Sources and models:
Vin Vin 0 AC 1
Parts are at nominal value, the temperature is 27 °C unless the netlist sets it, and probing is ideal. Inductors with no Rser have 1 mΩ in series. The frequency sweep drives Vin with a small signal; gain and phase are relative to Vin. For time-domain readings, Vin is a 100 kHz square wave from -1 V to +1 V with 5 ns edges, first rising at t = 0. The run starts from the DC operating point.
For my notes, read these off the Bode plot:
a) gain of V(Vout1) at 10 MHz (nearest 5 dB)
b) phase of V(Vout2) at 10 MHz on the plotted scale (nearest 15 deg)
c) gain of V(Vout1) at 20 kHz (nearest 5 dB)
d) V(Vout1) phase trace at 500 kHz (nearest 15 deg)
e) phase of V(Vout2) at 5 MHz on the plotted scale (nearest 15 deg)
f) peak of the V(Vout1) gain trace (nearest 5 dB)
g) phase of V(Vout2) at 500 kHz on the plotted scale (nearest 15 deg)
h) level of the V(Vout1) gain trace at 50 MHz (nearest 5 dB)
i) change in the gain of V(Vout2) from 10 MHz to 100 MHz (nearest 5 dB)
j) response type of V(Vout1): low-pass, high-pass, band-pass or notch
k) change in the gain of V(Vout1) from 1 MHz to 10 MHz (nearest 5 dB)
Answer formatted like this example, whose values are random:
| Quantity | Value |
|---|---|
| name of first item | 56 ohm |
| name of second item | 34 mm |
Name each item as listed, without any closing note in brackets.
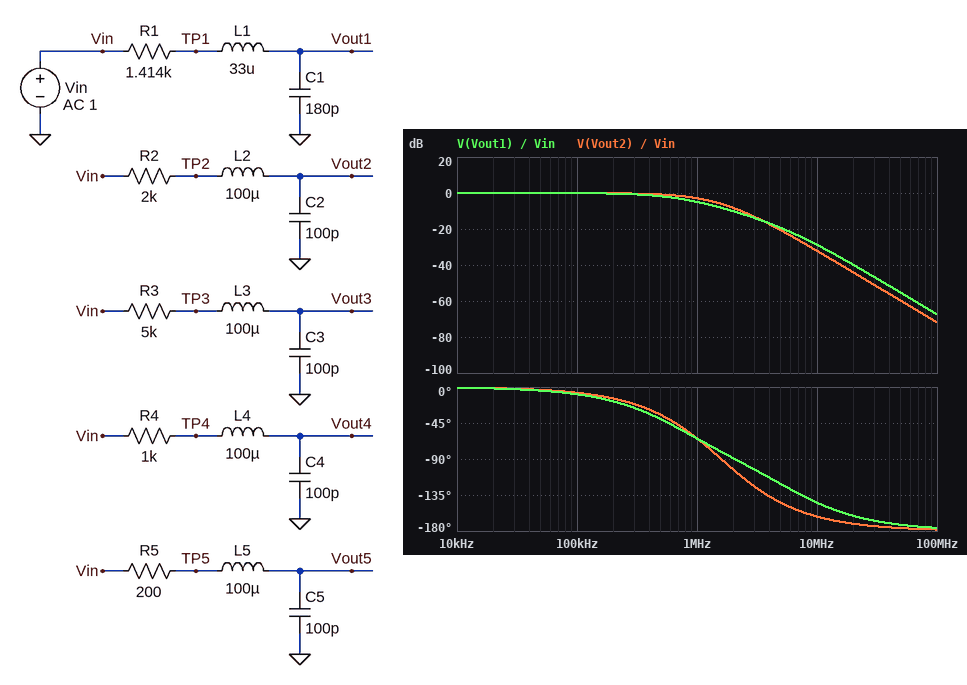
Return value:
| Quantity | Value |
|---|---|
| gain of V(Vout1) at 10 MHz | -30 dB |
| phase of V(Vout2) at 10 MHz on the plotted scale | -165 deg |
| gain of V(Vout1) at 20 kHz | 0 dB |
| V(Vout1) phase trace at 500 kHz | -45 deg |
| phase of V(Vout2) at 5 MHz on the plotted scale | -150 deg |
| peak of the V(Vout1) gain trace | 0 dB |
| phase of V(Vout2) at 500 kHz on the plotted scale | -30 deg |
| level of the V(Vout1) gain trace at 50 MHz | -55 dB |
| change in the gain of V(Vout2) from 10 MHz to 100 MHz | -40 dB |
| response type of V(Vout1): low-pass, high-pass, band-pass or notch | low-pass |
| change in the gain of V(Vout1) from 1 MHz to 10 MHz | -25 dB |
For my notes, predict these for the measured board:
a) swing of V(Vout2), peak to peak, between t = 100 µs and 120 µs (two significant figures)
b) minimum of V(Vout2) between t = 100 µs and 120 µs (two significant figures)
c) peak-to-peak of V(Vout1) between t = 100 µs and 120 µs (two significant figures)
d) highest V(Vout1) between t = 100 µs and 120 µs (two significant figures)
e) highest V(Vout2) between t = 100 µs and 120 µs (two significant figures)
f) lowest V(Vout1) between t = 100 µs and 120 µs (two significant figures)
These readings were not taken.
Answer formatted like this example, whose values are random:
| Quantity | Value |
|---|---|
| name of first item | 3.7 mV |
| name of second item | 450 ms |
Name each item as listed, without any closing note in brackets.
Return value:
| Quantity | Value |
|---|---|
| swing of V(Vout2), peak to peak, between t = 100 µs and 120 µs | 2.0 V |
| minimum of V(Vout2) between t = 100 µs and 120 µs | -1.0 V |
| peak-to-peak of V(Vout1) between t = 100 µs and 120 µs | 2.0 V |
| highest V(Vout1) between t = 100 µs and 120 µs | 1.0 V |
| highest V(Vout2) between t = 100 µs and 120 µs | 1.0 V |
| lowest V(Vout1) between t = 100 µs and 120 µs | -1.0 V |
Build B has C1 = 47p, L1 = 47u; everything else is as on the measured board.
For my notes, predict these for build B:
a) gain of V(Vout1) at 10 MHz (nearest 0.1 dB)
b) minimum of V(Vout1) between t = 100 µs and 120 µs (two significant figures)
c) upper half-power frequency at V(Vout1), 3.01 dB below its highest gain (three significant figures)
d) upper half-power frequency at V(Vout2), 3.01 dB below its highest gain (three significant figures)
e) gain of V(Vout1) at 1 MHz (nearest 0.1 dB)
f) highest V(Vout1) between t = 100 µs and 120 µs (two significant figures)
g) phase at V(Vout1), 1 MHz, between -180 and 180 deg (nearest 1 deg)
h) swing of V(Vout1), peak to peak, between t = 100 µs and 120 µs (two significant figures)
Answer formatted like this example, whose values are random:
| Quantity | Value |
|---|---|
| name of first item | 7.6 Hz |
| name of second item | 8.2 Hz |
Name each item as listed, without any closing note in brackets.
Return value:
| Quantity | Value |
|---|---|
| gain of V(Vout1) at 10 MHz | -18.9 dB |
| minimum of V(Vout1) between t = 100 µs and 120 µs | -1.1 V |
| upper half-power frequency at V(Vout1), 3.01 dB below its highest gain | 3.39 MHz |
| upper half-power frequency at V(Vout2), 3.01 dB below its highest gain | 1.02 MHz |
| gain of V(Vout1) at 1 MHz | 0 dB |
| highest V(Vout1) between t = 100 µs and 120 µs | 1.1 V |
| phase at V(Vout1), 1 MHz, between -180 and 180 deg | -25 deg |
| swing of V(Vout1), peak to peak, between t = 100 µs and 120 µs | 2.2 V |
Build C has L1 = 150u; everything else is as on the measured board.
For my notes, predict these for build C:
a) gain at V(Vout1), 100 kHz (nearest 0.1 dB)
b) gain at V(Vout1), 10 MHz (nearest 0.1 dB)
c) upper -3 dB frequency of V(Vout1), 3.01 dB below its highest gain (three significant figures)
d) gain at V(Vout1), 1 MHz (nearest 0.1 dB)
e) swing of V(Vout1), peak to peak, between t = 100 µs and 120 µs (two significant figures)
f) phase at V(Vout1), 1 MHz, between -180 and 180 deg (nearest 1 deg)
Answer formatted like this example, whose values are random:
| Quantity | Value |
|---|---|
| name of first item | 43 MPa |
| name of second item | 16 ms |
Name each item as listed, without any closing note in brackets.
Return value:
| Quantity | Value |
|---|---|
| gain at V(Vout1), 100 kHz | 0 dB |
| gain at V(Vout1), 10 MHz | -40.6 dB |
| upper -3 dB frequency of V(Vout1), 3.01 dB below its highest gain | 877 kHz |
| gain at V(Vout1), 1 MHz | -4.1 dB |
| swing of V(Vout1), peak to peak, between t = 100 µs and 120 µs | 2.1 V |
| phase at V(Vout1), 1 MHz, between -180 and 180 deg | -92 deg |
